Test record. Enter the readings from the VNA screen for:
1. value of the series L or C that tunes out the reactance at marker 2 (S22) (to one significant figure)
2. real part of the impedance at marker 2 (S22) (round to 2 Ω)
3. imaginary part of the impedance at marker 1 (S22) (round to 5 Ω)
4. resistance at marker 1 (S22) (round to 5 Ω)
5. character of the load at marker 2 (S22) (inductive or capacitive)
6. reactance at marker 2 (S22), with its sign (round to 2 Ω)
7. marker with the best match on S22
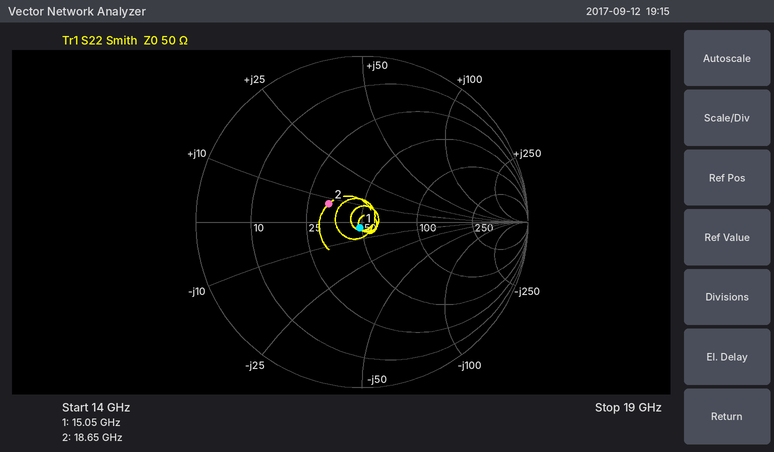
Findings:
1 pF
32 Ω
-5 Ω
50 Ω
inductive
+8 Ω
marker 1
